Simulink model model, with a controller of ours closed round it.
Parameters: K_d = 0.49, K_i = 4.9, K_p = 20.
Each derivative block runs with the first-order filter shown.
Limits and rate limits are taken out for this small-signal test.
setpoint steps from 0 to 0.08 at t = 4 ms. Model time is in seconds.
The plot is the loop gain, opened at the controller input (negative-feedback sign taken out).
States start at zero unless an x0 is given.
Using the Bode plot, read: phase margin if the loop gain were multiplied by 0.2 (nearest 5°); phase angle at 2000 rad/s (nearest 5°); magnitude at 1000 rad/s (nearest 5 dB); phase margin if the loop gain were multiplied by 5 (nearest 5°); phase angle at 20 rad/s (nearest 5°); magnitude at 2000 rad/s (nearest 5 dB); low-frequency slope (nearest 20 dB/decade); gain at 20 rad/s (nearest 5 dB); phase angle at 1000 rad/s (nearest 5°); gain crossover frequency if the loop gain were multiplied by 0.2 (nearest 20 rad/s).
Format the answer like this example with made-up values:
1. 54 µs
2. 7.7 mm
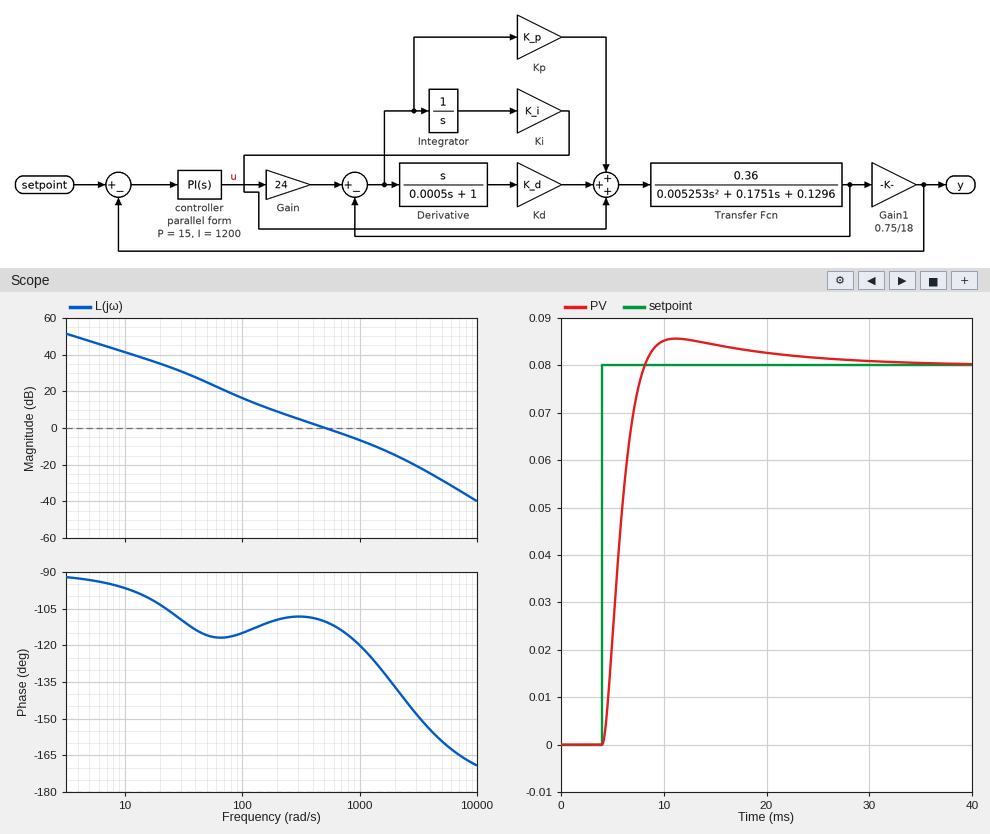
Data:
1. 65°
2. -135°
3. -5 dB
4. 45°
5. -105°
6. -15 dB
7. -20 dB/decade
8. 35 dB
9. -120°
10. 120 rad/s
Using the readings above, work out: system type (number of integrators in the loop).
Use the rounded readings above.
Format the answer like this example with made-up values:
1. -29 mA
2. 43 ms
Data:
1. 1
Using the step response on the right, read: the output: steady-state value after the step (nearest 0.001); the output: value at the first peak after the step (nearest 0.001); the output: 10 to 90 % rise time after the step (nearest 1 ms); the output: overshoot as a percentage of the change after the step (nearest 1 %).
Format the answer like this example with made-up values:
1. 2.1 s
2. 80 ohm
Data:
1. 0.080
2. 0.086
3. 3 ms
4. 7 %
